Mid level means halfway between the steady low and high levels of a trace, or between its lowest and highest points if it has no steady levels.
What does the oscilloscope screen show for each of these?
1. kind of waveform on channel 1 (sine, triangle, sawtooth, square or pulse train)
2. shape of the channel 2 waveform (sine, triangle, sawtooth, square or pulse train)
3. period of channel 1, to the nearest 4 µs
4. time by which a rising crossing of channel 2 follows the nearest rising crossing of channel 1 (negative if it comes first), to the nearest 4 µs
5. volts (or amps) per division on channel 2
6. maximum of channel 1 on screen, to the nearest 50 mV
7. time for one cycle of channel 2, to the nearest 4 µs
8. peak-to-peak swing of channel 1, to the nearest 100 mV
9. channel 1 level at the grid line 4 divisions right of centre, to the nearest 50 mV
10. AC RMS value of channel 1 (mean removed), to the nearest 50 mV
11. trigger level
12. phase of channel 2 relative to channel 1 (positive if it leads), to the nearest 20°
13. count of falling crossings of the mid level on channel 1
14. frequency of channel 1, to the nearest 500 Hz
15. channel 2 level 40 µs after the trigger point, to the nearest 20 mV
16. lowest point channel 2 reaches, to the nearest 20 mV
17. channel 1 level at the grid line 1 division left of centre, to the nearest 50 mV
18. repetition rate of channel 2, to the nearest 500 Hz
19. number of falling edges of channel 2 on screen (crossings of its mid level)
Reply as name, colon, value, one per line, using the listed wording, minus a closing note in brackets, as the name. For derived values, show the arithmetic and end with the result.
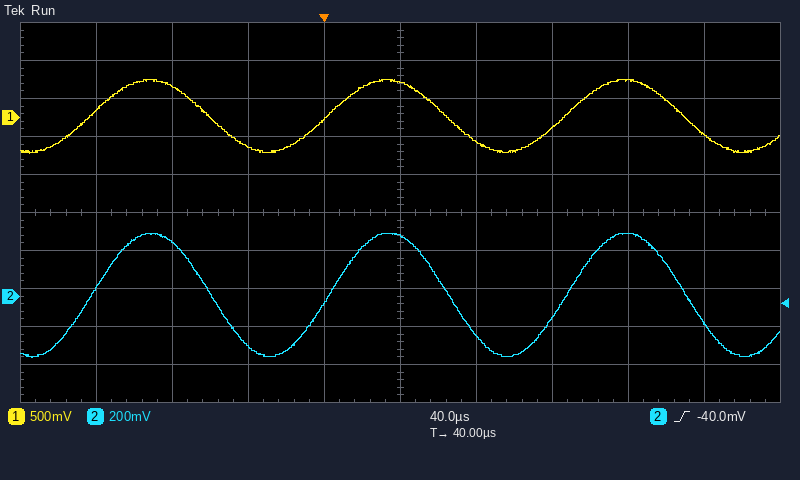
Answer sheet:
kind of waveform on channel 1: sine
shape of the channel 2 waveform: sine
period of channel 1, to the nearest 4 µs: 124 µs
time by which a rising crossing of channel 2 follows the nearest rising crossing of channel 1 (negative if it comes first), to the nearest 4 µs: 0 µs
volts (or amps) per division on channel 2: 200 mV
maximum of channel 1 on screen, to the nearest 50 mV: 500 mV
time for one cycle of channel 2, to the nearest 4 µs: 124 µs
peak-to-peak swing of channel 1, to the nearest 100 mV: 1.00 V
channel 1 level at the grid line 4 divisions right of centre, to the nearest 50 mV: -200 mV
AC RMS value of channel 1 (mean removed), to the nearest 50 mV: 1.00 V / (2√2) ≈ 354 mV, so 350 mV to the nearest 50 mV
trigger level: -40.0 mV
phase of channel 2 relative to channel 1 (positive if it leads), to the nearest 20°: −360° × (0 µs) / 124 µs ≈ 0°
count of falling crossings of the mid level on channel 1: 3
frequency of channel 1, to the nearest 500 Hz: 1 / 124 µs ≈ 8.06 kHz, so 8.0 kHz to the nearest 500 Hz
channel 2 level 40 µs after the trigger point, to the nearest 20 mV: 320 mV
lowest point channel 2 reaches, to the nearest 20 mV: -320 mV
channel 1 level at the grid line 1 division left of centre, to the nearest 50 mV: 0 mV
repetition rate of channel 2, to the nearest 500 Hz: 1 / 124 µs ≈ 8.06 kHz, so 8.0 kHz to the nearest 500 Hz
number of falling edges of channel 2 on screen: 3
